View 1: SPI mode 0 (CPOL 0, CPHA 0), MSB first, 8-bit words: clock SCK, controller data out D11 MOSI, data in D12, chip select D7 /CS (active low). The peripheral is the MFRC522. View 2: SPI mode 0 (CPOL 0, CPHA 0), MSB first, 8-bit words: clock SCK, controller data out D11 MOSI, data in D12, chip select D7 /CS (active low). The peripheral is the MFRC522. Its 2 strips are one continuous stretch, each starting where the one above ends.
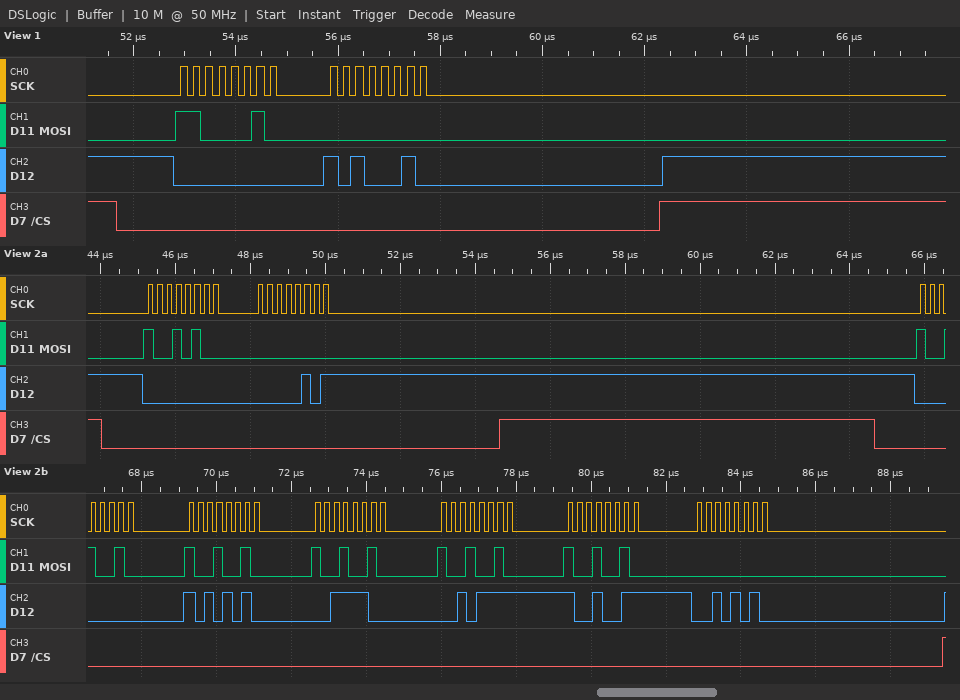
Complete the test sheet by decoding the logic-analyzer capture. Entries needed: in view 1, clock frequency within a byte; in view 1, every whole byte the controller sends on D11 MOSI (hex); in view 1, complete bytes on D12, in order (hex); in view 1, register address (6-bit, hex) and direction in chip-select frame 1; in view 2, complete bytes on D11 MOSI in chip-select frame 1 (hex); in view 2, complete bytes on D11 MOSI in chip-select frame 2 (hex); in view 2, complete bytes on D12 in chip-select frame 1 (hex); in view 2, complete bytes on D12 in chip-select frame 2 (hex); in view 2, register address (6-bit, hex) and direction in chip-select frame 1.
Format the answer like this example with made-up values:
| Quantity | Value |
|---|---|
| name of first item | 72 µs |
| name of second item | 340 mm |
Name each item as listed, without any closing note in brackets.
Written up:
| Quantity | Value |
|---|---|
| in view 1, clock frequency within a byte | 4 MHz |
| in view 1, every whole byte the controller sends on D11 MOSI | 0xC2 0x00 |
| in view 1, complete bytes on D12, in order | 0x00 0xA2 |
| in view 1, register address (6-bit, hex) and direction in chip-select frame 1 | 0x21 read |
| in view 2, complete bytes on D11 MOSI in chip-select frame 1 | 0x94 0x00 |
| in view 2, complete bytes on D11 MOSI in chip-select frame 2 | 0x92 0x92 0x92 0x92 0x92 0x00 |
| in view 2, complete bytes on D12 in chip-select frame 1 | 0x00 0x05 |
| in view 2, complete bytes on D12 in chip-select frame 2 | 0x00 0xAA 0x3C 0x2F 0x93 0x2A |
| in view 2, register address (6-bit, hex) and direction in chip-select frame 1 | 0x0A read |
